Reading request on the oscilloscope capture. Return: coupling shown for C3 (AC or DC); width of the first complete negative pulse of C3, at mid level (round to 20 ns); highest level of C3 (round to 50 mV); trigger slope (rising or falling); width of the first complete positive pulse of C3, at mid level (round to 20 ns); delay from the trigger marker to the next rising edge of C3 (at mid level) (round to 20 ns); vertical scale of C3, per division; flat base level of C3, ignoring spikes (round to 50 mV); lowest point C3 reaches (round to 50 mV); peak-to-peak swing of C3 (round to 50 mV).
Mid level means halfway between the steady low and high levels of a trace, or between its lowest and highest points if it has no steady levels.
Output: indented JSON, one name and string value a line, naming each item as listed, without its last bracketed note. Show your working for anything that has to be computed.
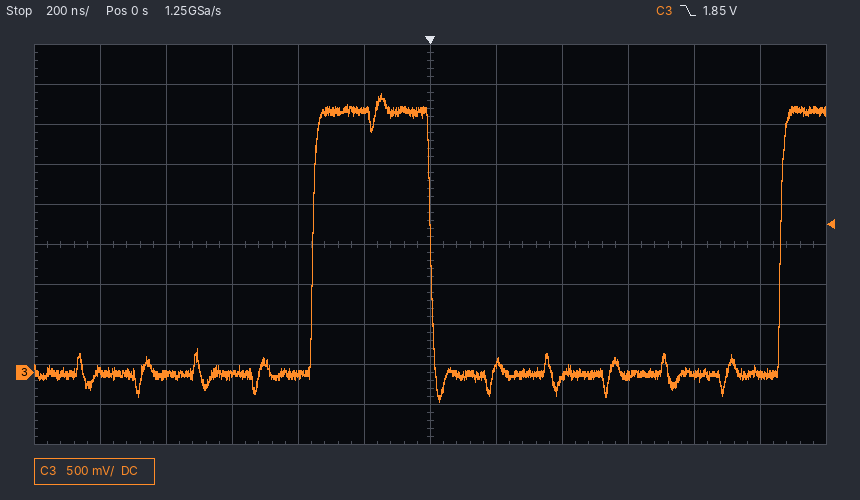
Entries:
{
  "coupling shown for C3": "DC",
  "width of the first complete negative pulse of C3, at mid level": "1.06 µs",
  "highest level of C3": "3.50 V",
  "trigger slope": "falling",
  "width of the first complete positive pulse of C3, at mid level": "360 ns",
  "delay from the trigger marker to the next rising edge of C3 (at mid level)": "1.06 µs",
  "vertical scale of C3, per division": "500 mV",
  "flat base level of C3, ignoring spikes": "0 mV",
  "lowest point C3 reaches": "-350 mV",
  "peak-to-peak swing of C3": "3.50 V − (-350 mV) = 3.85 V"
}
